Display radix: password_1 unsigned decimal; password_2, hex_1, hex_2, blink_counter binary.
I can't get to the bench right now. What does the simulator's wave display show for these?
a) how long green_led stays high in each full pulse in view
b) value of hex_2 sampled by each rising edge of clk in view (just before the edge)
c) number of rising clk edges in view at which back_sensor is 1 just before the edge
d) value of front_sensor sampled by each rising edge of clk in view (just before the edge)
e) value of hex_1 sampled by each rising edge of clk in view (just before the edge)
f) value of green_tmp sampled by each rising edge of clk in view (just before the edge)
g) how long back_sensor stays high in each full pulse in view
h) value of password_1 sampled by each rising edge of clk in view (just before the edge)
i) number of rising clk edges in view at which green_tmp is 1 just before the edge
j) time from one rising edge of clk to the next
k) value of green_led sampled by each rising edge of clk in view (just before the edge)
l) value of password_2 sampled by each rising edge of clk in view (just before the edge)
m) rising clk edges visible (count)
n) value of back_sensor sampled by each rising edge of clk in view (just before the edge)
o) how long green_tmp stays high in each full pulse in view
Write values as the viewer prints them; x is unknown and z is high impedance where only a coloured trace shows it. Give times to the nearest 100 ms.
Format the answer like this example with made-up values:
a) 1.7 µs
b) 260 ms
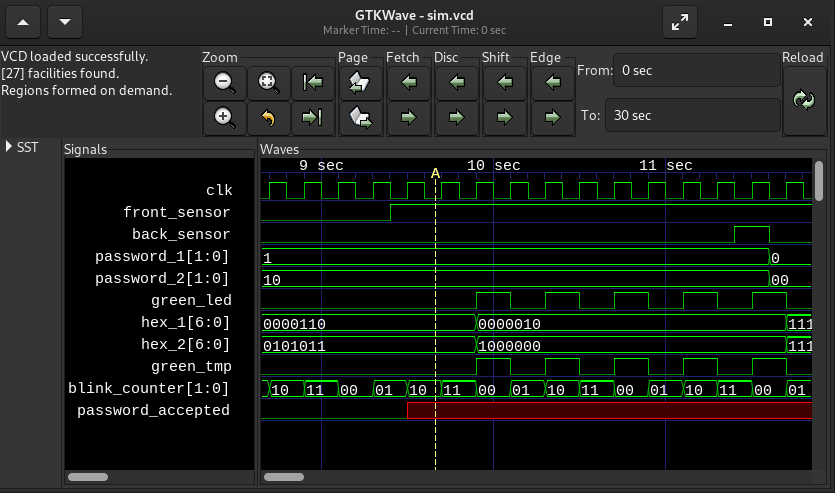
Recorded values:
a) 200 ms, 200 ms, 200 ms, 200 ms, 200 ms
b) 0101011, 0101011, 0101011, 0101011, 0101011, 0101011, 0101011, 1000000, 1000000, 1000000, 1000000, 1000000, 1000000, 1000000, 1000000, 1000000
c) 1
d) 0 0 0 0 1 1 1 1 1 1 1 1 1 1 1 1
e) 0000110, 0000110, 0000110, 0000110, 0000110, 0000110, 0000110, 0000010, 0000010, 0000010, 0000010, 0000010, 0000010, 0000010, 0000010, 0000010
f) 0 0 0 0 0 0 0 1 0 1 0 1 0 1 0 1
g) 200 ms
h) 1, 1, 1, 1, 1, 1, 1, 1, 1, 1, 1, 1, 1, 1, 1, 0
i) 5
j) 200 ms
k) 0 0 0 0 0 0 0 1 0 1 0 1 0 1 0 1
l) 10, 10, 10, 10, 10, 10, 10, 10, 10, 10, 10, 10, 10, 10, 10, 00
m) 16
n) 0 0 0 0 0 0 0 0 0 0 0 0 0 0 1 0
o) 200 ms, 200 ms, 200 ms, 200 ms, 200 ms
